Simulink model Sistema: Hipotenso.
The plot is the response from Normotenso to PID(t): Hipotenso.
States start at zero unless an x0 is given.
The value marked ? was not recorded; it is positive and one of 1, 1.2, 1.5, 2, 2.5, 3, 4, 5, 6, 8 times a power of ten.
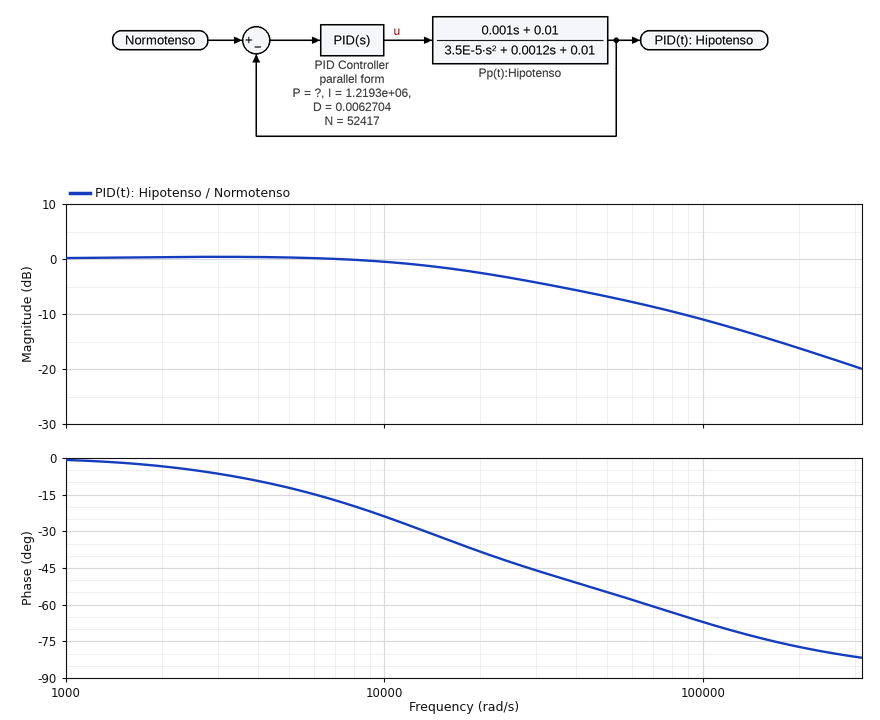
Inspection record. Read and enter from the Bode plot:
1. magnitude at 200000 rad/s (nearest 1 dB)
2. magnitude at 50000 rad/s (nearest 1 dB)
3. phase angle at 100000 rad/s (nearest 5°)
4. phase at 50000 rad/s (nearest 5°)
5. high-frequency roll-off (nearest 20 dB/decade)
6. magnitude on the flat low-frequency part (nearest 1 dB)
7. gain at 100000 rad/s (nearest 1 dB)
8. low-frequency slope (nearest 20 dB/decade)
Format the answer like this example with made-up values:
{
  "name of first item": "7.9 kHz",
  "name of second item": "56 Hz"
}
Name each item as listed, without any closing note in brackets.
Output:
{
  "magnitude at 200000 rad/s": "-16 dB",
  "magnitude at 50000 rad/s": "-7 dB",
  "phase angle at 100000 rad/s": "-65°",
  "phase at 50000 rad/s": "-55°",
  "high-frequency roll-off": "-20 dB/decade",
  "magnitude on the flat low-frequency part": "0 dB",
  "gain at 100000 rad/s": "-11 dB",
  "low-frequency slope": "0 dB/decade"
}
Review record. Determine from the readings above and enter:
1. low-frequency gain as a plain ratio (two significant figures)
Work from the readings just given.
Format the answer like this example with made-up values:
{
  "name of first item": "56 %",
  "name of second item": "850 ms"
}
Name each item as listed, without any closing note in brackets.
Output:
{
  "low-frequency gain as a plain ratio": "1.0"
}
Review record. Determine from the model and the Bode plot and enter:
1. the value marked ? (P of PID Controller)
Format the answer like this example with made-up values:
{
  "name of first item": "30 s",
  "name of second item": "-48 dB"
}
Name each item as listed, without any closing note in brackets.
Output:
{
  "the value marked ?": "800"
}
